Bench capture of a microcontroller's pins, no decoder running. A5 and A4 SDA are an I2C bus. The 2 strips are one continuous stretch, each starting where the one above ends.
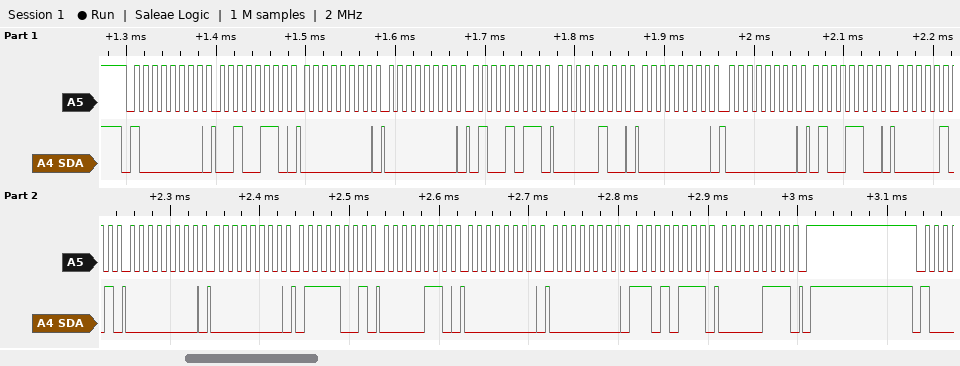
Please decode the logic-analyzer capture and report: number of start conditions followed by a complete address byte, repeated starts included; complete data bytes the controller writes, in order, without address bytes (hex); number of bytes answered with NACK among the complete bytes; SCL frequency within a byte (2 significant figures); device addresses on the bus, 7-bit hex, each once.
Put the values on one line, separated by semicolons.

1; 26 00 00 4B 04 00 00 4C 05 00 00 79 06 00 00 D7 07; 0; 100 kHz; 0x40
